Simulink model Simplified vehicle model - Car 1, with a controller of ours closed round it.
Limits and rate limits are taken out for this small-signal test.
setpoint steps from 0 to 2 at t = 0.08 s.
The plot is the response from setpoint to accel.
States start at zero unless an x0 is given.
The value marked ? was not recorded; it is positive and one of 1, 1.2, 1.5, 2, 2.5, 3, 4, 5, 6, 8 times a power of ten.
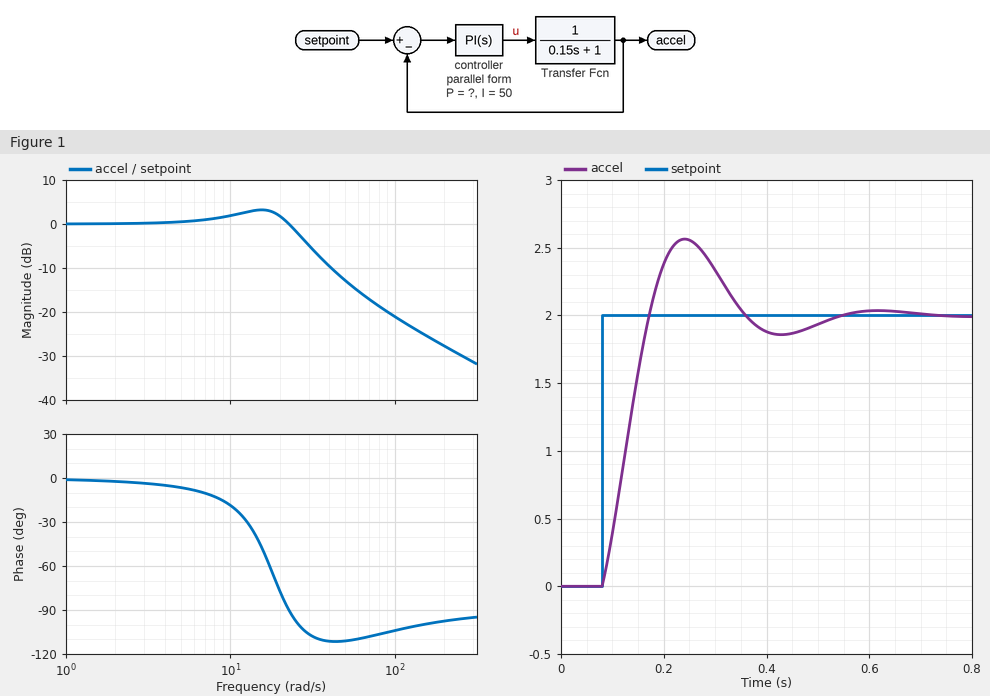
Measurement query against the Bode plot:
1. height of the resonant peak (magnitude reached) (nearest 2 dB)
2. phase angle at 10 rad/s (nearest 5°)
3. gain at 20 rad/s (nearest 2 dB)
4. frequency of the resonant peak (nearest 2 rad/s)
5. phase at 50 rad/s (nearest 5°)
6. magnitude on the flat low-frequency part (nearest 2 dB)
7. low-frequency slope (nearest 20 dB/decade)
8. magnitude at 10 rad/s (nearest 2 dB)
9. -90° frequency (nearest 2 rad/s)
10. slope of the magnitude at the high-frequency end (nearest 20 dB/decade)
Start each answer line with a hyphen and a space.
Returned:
- 4 dB
- -20°
- 2 dB
- 16 rad/s
- -110°
- 0 dB
- 0 dB/decade
- 2 dB
- 22 rad/s
- -20 dB/decade
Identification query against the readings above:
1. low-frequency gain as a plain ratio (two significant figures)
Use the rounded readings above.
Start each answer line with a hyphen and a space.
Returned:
- 1.0
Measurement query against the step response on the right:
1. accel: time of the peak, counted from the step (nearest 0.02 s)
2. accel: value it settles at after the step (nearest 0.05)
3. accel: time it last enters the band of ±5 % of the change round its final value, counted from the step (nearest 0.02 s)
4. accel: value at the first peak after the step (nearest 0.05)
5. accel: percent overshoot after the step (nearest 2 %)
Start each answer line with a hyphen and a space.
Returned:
- 0.16 s
- 2.00
- 0.40 s
- 2.55
- 28 %
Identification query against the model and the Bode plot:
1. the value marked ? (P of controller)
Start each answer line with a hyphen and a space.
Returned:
- 1.2
